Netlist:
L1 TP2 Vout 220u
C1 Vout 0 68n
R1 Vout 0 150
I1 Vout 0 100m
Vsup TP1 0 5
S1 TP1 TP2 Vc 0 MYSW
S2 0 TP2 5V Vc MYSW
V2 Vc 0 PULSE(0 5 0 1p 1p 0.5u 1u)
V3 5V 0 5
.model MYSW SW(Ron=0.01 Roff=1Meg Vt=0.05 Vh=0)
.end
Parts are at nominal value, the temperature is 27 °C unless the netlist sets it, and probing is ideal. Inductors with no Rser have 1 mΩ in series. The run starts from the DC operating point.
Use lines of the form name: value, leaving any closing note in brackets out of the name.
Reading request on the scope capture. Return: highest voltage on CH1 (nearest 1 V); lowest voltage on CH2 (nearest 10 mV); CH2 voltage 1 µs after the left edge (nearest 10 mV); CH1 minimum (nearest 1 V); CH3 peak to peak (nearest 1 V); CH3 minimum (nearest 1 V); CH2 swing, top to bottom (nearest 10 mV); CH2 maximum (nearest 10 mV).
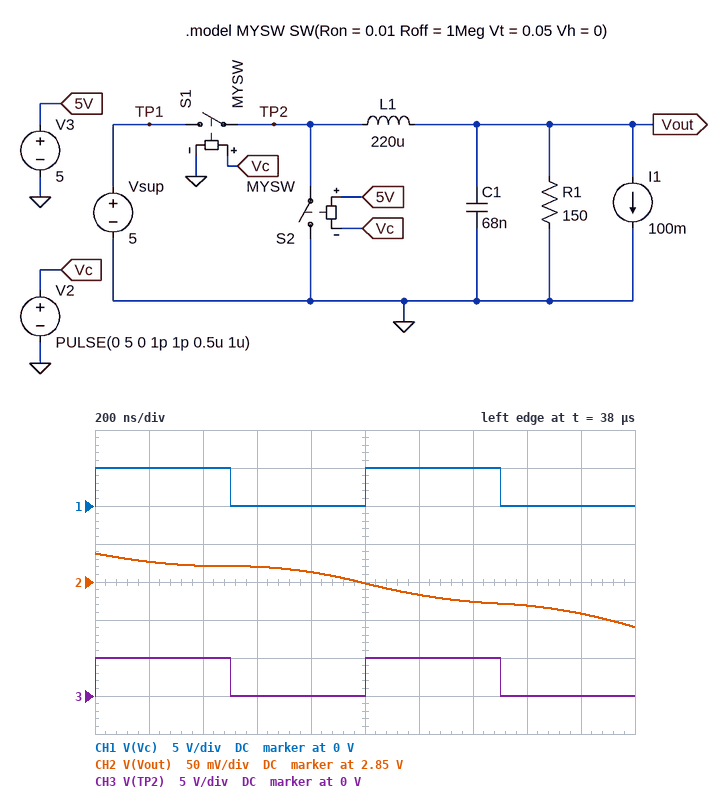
highest voltage on CH1: 5 V
lowest voltage on CH2: 2.79 V
CH2 voltage 1 µs after the left edge: 2.85 V
CH1 minimum: 0 V
CH3 peak to peak: 5 V
CH3 minimum: 0 V
CH2 swing, top to bottom: 100 mV
CH2 maximum: 2.89 V
